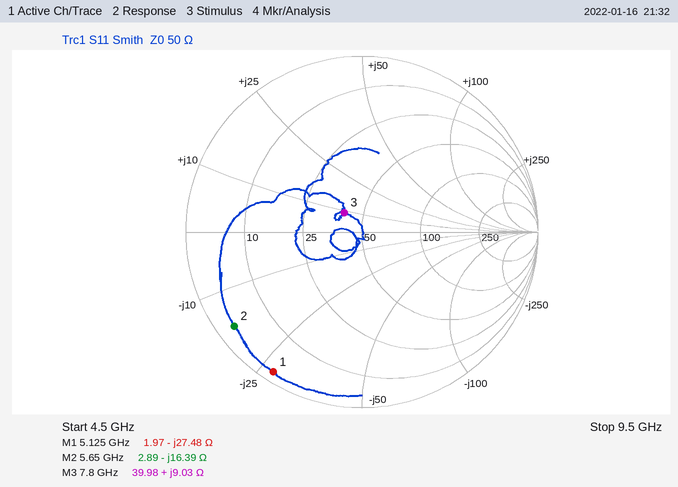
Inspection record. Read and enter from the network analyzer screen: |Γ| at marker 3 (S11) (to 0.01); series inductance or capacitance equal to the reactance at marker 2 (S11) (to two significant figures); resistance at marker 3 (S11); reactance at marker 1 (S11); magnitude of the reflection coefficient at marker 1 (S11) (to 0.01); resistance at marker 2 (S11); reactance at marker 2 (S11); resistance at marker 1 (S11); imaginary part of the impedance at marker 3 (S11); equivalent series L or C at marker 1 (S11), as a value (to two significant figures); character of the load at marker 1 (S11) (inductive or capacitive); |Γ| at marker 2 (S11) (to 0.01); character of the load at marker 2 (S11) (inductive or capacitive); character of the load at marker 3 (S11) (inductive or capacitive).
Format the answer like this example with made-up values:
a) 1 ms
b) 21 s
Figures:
a) 0.15
b) 1.7 pF
c) 39.98 Ω
d) -27.48 Ω
e) 0.94
f) 2.89 Ω
g) -16.39 Ω
h) 1.97 Ω
i) +9.03 Ω
j) 1.1 pF
k) capacitive
l) 0.90
m) capacitive
n) inductive
